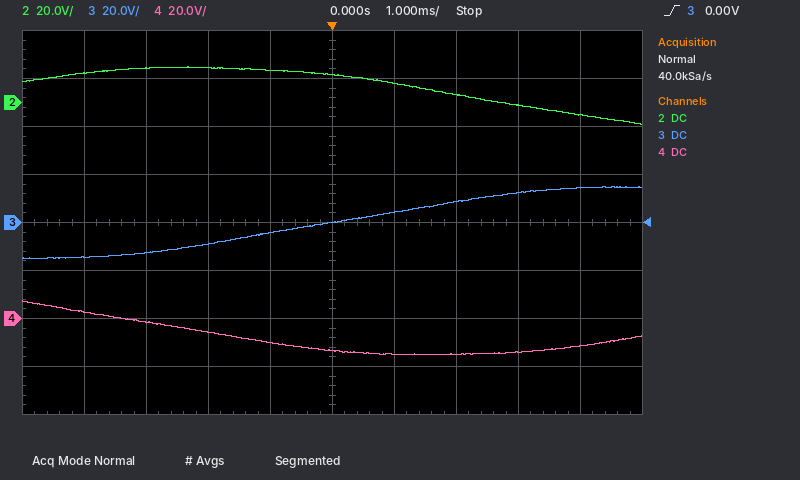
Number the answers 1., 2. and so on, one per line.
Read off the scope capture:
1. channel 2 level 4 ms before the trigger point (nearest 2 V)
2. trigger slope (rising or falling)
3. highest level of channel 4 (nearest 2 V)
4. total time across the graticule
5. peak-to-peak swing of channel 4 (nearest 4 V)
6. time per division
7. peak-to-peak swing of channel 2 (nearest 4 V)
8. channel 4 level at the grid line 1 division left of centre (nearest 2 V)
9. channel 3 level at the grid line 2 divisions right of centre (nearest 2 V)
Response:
1. 12 V
2. rising
3. 8 V
4. 10 ms
5. 24 V
6. 1 ms
7. 24 V
8. -10 V
9. 8 V
